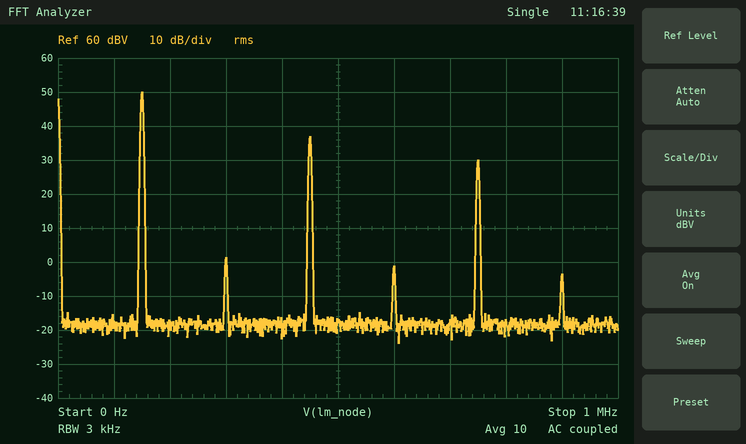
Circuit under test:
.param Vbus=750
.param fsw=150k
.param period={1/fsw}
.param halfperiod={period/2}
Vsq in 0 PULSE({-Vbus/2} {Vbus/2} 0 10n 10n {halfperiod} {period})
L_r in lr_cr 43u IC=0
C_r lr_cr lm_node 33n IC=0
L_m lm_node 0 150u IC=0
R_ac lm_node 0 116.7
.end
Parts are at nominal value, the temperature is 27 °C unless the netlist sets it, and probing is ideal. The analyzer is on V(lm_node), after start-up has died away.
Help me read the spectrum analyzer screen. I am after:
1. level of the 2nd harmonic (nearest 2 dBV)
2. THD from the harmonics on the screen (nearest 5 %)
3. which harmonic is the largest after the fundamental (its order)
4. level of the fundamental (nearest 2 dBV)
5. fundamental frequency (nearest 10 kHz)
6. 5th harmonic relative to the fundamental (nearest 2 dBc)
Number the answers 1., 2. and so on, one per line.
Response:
1. 2 dBV
2. 25 %
3. 3
4. 50 dBV
5. 150 kHz
6. -20 dBc
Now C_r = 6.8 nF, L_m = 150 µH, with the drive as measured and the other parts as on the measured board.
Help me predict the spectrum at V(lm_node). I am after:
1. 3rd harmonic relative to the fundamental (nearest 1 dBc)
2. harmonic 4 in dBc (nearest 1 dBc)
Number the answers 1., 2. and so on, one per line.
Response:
1. -12 dBc
2. -51 dBc
